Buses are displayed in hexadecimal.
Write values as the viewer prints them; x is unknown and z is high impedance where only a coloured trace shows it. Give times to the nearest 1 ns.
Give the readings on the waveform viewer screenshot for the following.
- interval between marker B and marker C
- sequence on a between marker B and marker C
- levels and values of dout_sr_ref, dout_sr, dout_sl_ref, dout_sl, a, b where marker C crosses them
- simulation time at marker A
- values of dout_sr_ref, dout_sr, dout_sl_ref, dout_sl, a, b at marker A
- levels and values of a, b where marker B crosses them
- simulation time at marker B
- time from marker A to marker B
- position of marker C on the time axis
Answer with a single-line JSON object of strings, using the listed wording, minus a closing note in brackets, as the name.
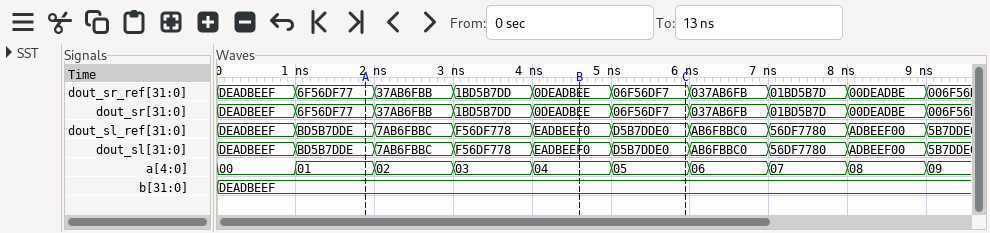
{"interval between marker B and marker C": "1 ns", "sequence on a between marker B and marker C": "04, 05", "levels and values of dout_sr_ref, dout_sr, dout_sl_ref, dout_sl, a, b where marker C crosses them": "dout_sr_ref=06F56DF7, dout_sr=06F56DF7, dout_sl_ref=D5B7DDE0, dout_sl=D5B7DDE0, a=05, b=DEADBEEF", "simulation time at marker A": "2 ns", "values of dout_sr_ref, dout_sr, dout_sl_ref, dout_sl, a, b at marker A": "dout_sr_ref=6F56DF77, dout_sr=6F56DF77, dout_sl_ref=BD5B7DDE, dout_sl=BD5B7DDE, a=01, b=DEADBEEF", "levels and values of a, b where marker B crosses them": "a=04, b=DEADBEEF", "simulation time at marker B": "5 ns", "time from marker A to marker B": "3 ns", "position of marker C on the time axis": "6 ns"}
